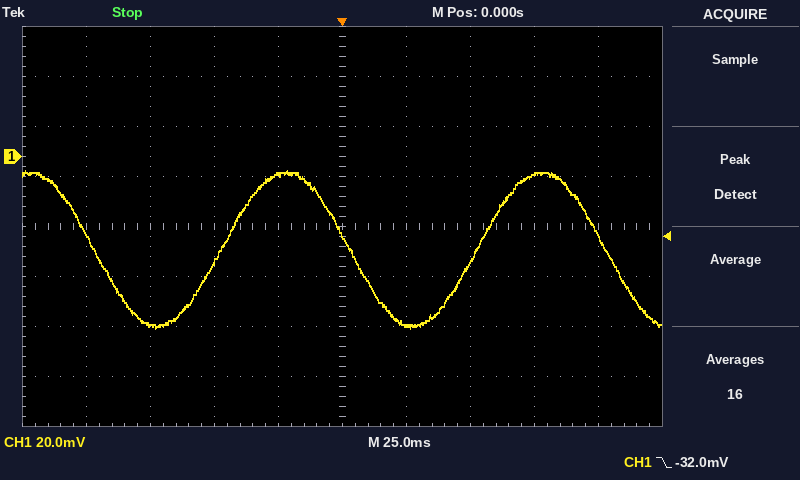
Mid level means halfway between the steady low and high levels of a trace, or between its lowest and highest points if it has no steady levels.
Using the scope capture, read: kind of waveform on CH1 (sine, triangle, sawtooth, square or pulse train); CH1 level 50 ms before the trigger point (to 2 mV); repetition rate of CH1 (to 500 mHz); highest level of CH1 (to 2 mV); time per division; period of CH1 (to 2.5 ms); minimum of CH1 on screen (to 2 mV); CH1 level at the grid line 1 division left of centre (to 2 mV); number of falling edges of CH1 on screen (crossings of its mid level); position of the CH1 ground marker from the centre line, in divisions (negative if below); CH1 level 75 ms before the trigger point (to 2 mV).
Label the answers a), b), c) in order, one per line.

a) sine
b) -42 mV
c) 10.0 Hz
d) -6 mV
e) 25 ms
f) 100.0 ms
g) -68 mV
h) -8 mV
i) 3
j) +1.4 div
k) -68 mV
